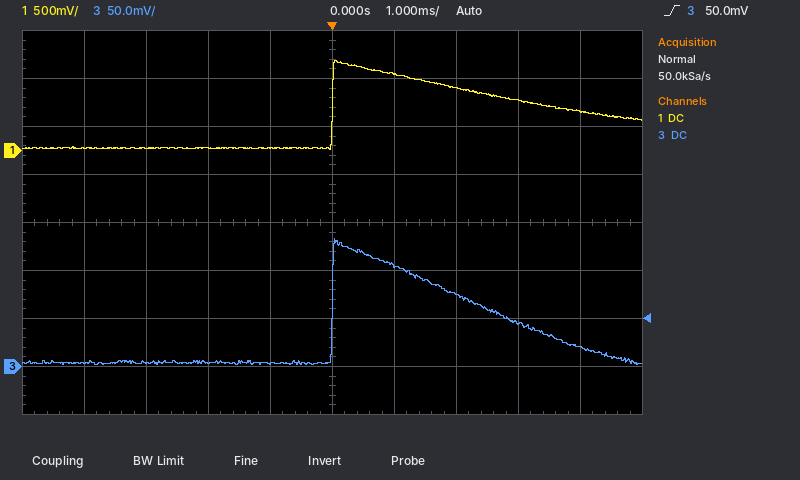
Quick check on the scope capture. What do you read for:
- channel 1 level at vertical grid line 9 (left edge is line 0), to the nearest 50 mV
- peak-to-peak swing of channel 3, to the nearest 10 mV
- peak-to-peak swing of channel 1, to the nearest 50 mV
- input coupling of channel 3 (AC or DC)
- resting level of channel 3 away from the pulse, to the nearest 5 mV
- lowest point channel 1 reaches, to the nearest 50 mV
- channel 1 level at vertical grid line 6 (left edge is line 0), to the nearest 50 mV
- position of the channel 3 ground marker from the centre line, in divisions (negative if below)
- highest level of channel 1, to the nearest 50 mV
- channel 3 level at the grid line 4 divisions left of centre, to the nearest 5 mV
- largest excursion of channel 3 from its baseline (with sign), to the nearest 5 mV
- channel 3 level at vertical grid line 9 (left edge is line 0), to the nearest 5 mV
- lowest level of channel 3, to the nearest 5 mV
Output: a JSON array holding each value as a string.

["400 mV", "130 mV", "950 mV", "DC", "5 mV", "0 mV", "800 mV", "-3.0 div", "950 mV", "5 mV", "+130 mV", "20 mV", "0 mV"]
